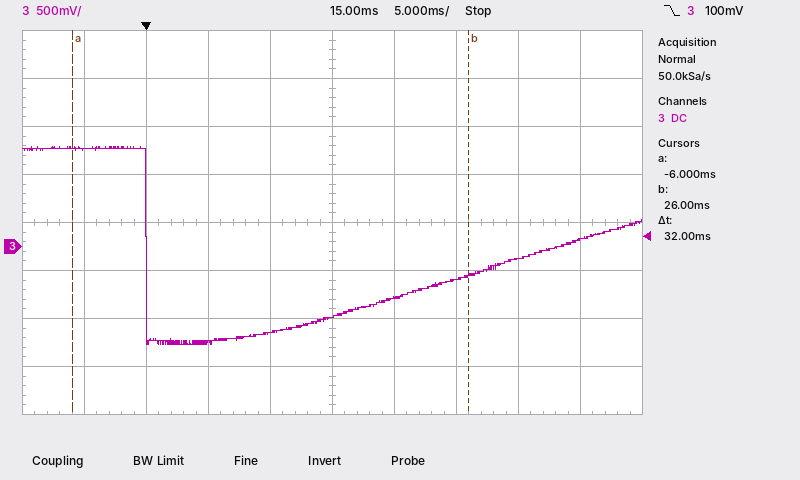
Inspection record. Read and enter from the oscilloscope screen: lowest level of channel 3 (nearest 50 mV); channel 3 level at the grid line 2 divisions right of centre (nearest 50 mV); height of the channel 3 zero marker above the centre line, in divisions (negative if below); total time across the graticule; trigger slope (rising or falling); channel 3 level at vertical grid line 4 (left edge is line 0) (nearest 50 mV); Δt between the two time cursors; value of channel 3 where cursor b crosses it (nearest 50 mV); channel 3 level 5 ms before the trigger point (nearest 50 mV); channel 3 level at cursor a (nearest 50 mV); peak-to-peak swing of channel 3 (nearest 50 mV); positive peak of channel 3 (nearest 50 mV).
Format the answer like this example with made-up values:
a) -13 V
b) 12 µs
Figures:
a) -1.00 V
b) -350 mV
c) -0.5 div
d) 50 ms
e) falling
f) -900 mV
g) 32 ms
h) -300 mV
i) 1.00 V
j) 1.00 V
k) 2.05 V
l) 1.05 V
